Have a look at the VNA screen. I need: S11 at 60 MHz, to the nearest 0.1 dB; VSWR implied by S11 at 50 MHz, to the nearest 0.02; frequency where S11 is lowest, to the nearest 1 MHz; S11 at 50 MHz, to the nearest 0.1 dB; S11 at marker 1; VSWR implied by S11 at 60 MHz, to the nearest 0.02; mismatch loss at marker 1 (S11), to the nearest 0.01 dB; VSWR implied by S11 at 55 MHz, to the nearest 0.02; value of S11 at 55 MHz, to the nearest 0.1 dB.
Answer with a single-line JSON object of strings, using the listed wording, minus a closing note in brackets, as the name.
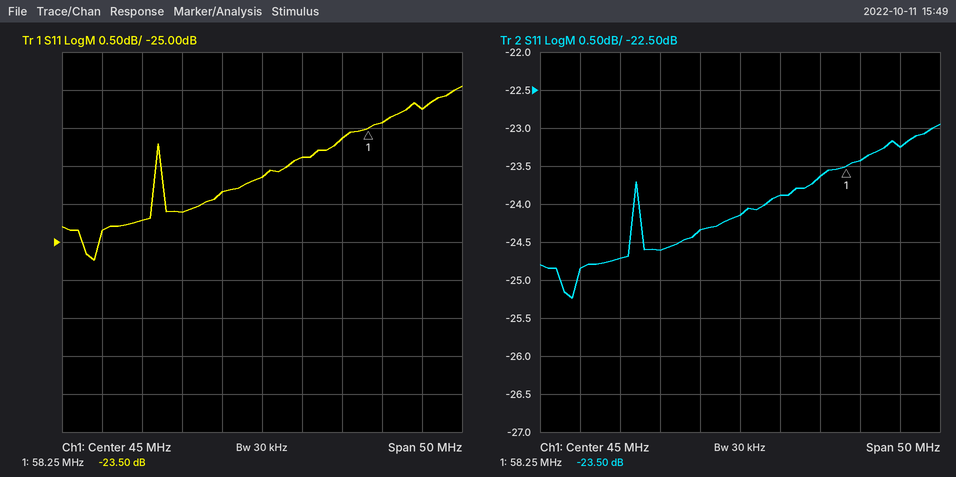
{"S11 at 60 MHz, to the nearest 0.1 dB": "-23.4 dB", "VSWR implied by S11 at 50 MHz, to the nearest 0.02": "1.14", "frequency where S11 is lowest, to the nearest 1 MHz": "24 MHz", "S11 at 50 MHz, to the nearest 0.1 dB": "-23.9 dB", "S11 at marker 1": "-23.50 dB", "VSWR implied by S11 at 60 MHz, to the nearest 0.02": "1.14", "mismatch loss at marker 1 (S11), to the nearest 0.01 dB": "0.02 dB", "VSWR implied by S11 at 55 MHz, to the nearest 0.02": "1.14", "value of S11 at 55 MHz, to the nearest 0.1 dB": "-23.6 dB"}
